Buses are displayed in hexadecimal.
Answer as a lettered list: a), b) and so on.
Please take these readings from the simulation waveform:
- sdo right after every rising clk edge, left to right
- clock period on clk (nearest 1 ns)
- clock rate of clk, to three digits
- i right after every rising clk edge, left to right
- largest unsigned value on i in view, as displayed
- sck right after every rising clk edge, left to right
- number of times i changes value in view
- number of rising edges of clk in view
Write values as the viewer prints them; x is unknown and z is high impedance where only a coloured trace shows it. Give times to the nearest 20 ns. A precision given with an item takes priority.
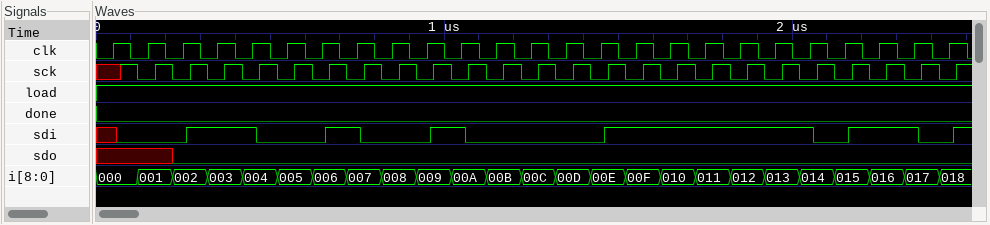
a) x x 0 0 0 0 0 0 0 0 0 0 0 0 0 0 0 0 0 0 0 0 0 0 0
b) 100 ns
c) 10.0 MHz
d) 000, 001, 002, 003, 004, 005, 006, 007, 008, 009, 00A, 00B, 00C, 00D, 00E, 00F, 010, 011, 012, 013, 014, 015, 016, 017, 018
e) 018
f) x 0 0 0 0 0 0 0 0 0 0 0 0 0 0 0 0 0 0 0 0 0 0 0 0
g) 24
h) 25
